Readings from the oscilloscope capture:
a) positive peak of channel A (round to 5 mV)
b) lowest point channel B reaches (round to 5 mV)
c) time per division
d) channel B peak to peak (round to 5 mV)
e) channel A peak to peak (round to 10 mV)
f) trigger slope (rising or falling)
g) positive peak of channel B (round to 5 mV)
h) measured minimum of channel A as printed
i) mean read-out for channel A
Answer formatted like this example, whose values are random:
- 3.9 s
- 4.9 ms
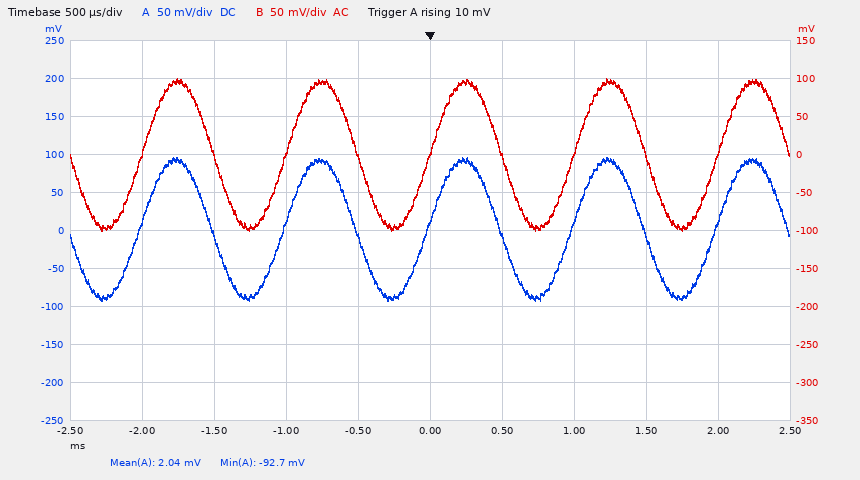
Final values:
- 95 mV
- -100 mV
- 500 µs
- 200 mV
- 190 mV
- rising
- 100 mV
- -92.7 mV
- 2.04 mV
